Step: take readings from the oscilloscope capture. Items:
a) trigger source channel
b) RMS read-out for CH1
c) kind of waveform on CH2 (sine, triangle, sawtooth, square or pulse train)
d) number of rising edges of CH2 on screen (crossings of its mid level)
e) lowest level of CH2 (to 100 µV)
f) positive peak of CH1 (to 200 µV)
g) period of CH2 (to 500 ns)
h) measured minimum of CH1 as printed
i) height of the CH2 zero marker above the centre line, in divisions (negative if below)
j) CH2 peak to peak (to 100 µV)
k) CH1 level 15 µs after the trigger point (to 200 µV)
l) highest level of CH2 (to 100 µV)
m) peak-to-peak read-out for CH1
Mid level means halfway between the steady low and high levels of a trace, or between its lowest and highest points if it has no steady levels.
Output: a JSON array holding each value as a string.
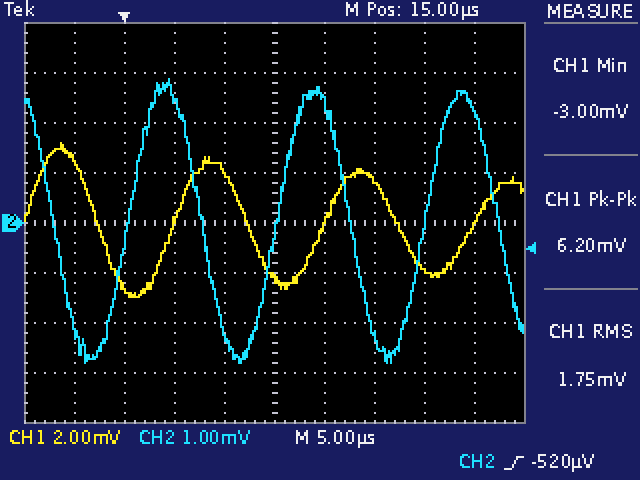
["CH2", "1.75 mV", "sine", "3", "-2.8 mV", "3.2 mV", "15.0 µs", "-3.00 mV", "0.0 div", "5.7 mV", "-2.2 mV", "2.9 mV", "6.20 mV"]
